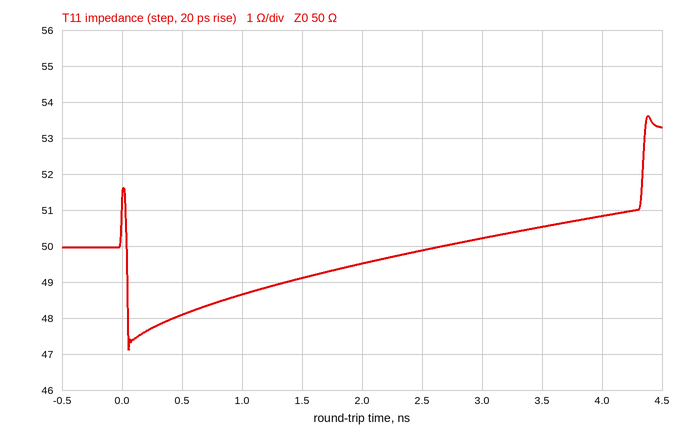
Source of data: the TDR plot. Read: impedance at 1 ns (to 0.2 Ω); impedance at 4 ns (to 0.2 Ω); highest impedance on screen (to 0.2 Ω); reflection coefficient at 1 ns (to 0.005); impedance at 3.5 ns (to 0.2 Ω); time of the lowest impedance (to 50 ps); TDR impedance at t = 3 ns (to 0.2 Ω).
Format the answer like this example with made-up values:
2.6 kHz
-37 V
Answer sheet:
48.6 Ω
50.8 Ω
53.6 Ω
-0.015
50.6 Ω
50 ps
50.2 Ω
